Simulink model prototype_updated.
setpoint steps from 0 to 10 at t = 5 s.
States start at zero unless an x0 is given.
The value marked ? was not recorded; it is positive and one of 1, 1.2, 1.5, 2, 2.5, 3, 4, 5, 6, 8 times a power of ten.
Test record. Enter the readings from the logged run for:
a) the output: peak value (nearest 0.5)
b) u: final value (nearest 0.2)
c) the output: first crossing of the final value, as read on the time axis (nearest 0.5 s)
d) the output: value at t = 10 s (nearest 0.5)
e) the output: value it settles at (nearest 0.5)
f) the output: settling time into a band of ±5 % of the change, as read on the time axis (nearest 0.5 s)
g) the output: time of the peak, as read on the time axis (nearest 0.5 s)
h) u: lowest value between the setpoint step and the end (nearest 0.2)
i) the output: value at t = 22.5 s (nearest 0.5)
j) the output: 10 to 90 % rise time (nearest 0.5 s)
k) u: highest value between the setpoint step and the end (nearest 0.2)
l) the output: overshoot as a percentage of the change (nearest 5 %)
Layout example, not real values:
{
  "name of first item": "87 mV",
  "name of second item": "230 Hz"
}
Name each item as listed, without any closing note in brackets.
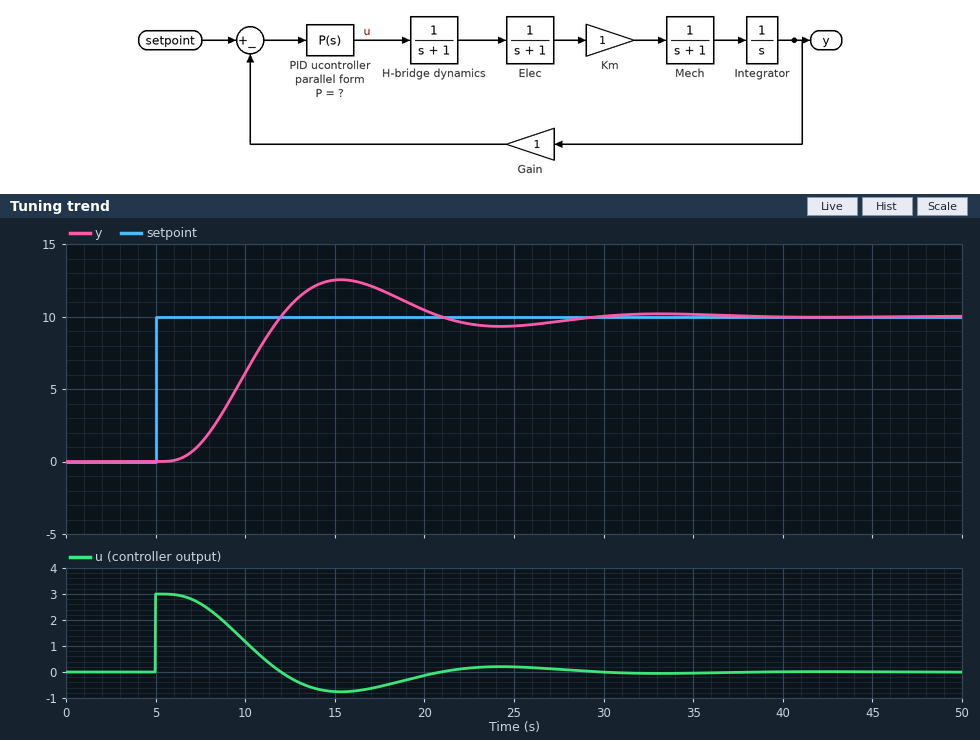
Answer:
{
  "the output: peak value": "12.5",
  "u: final value": "0.0",
  "the output: first crossing of the final value, as read on the time axis": "12.0 s",
  "the output: value at t = 10 s": "6.0",
  "the output: value it settles at": "10.0",
  "the output: settling time into a band of ±5 % of the change, as read on the time axis": "26.5 s",
  "the output: time of the peak, as read on the time axis": "15.5 s",
  "u: lowest value between the setpoint step and the end": "-0.8",
  "the output: value at t = 22.5 s": "9.5",
  "the output: 10 to 90 % rise time": "4.0 s",
  "u: highest value between the setpoint step and the end": "3.0",
  "the output: overshoot as a percentage of the change": "25 %"
}
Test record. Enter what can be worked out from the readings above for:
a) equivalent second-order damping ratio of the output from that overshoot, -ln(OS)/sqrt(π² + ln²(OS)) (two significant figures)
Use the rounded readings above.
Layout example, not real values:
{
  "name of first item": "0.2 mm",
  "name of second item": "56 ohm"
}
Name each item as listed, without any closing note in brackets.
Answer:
{
  "equivalent second-order damping ratio of the output from that overshoot, -ln(OS)/sqrt(π² + ln²(OS))": "0.40"
}
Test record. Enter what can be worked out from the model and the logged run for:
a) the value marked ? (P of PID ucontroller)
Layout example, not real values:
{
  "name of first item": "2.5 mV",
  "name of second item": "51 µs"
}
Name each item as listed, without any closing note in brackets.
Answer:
{
  "the value marked ?": "0.3"
}
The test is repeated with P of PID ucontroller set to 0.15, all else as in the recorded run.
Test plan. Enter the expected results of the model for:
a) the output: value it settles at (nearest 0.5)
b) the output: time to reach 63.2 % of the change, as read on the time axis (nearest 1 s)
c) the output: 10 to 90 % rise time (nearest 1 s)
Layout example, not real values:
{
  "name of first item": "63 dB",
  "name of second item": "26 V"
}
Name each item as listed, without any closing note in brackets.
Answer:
{
  "the output: value it settles at": "10.0",
  "the output: time to reach 63.2 % of the change, as read on the time axis": "13 s",
  "the output: 10 to 90 % rise time": "8 s"
}
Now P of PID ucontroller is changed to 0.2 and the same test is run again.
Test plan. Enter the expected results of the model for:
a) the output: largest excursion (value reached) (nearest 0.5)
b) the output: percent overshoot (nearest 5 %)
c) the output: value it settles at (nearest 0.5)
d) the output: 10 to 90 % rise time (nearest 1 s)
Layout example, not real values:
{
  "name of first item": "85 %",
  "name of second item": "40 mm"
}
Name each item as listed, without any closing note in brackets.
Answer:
{
  "the output: largest excursion (value reached)": "11.0",
  "the output: percent overshoot": "10 %",
  "the output: value it settles at": "10.0",
  "the output: 10 to 90 % rise time": "6 s"
}
